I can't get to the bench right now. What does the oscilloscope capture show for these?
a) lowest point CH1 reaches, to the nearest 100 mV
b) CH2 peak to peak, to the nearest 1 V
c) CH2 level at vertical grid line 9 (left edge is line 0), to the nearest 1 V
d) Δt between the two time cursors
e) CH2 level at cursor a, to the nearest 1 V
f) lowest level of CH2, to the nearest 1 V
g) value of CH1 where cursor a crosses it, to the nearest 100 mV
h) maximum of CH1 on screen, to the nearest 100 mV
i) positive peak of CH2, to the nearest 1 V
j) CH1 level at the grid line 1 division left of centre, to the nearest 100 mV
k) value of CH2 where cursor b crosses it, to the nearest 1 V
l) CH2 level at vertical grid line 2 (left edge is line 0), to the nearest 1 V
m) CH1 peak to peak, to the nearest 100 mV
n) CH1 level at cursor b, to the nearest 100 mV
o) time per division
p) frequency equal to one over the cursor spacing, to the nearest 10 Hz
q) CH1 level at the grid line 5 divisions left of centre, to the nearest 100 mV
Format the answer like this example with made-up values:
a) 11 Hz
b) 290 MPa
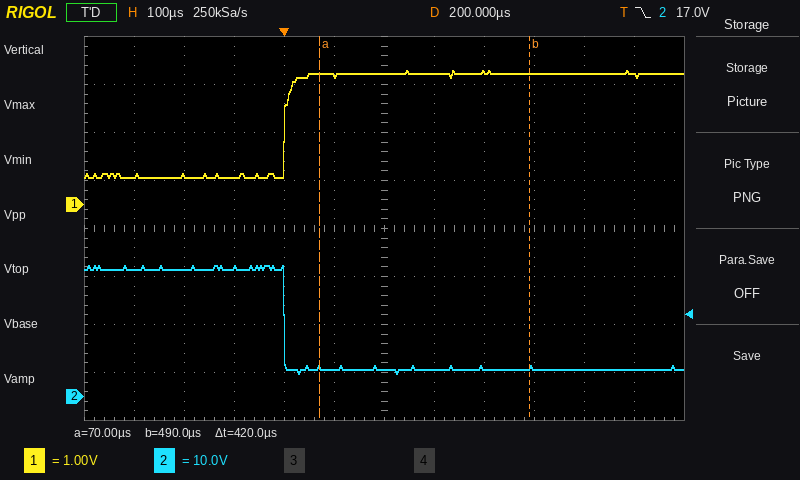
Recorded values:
a) 600 mV
b) 22 V
c) 6 V
d) 420 µs
e) 6 V
f) 5 V
g) 2.7 V
h) 2.8 V
i) 27 V
j) 2.7 V
k) 6 V
l) 26 V
m) 2.2 V
n) 2.7 V
o) 100 µs
p) 2.38 kHz
q) 600 mV
